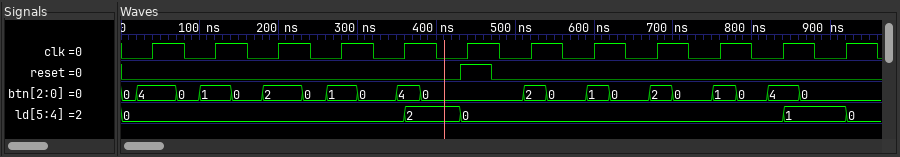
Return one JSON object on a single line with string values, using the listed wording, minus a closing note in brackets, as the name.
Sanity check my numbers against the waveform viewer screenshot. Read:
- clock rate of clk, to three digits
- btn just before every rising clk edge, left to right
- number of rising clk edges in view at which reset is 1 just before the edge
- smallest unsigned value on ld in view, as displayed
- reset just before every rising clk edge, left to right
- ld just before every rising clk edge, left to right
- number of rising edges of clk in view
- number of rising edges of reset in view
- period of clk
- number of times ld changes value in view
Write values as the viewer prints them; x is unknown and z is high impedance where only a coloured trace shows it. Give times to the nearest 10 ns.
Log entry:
{"clock rate of clk, to three digits": "12.5 MHz", "btn just before every rising clk edge, left to right": "4, 1, 2, 1, 4, 0, 2, 1, 2, 1, 4, 0", "number of rising clk edges in view at which reset is 1 just before the edge": "1", "smallest unsigned value on ld in view, as displayed": "0", "reset just before every rising clk edge, left to right": "0 0 0 0 0 1 0 0 0 0 0 0", "ld just before every rising clk edge, left to right": "0, 0, 0, 0, 0, 0, 0, 0, 0, 0, 0, 1", "number of rising edges of clk in view": "12", "number of rising edges of reset in view": "1", "period of clk": "80 ns", "number of times ld changes value in view": "4"}
